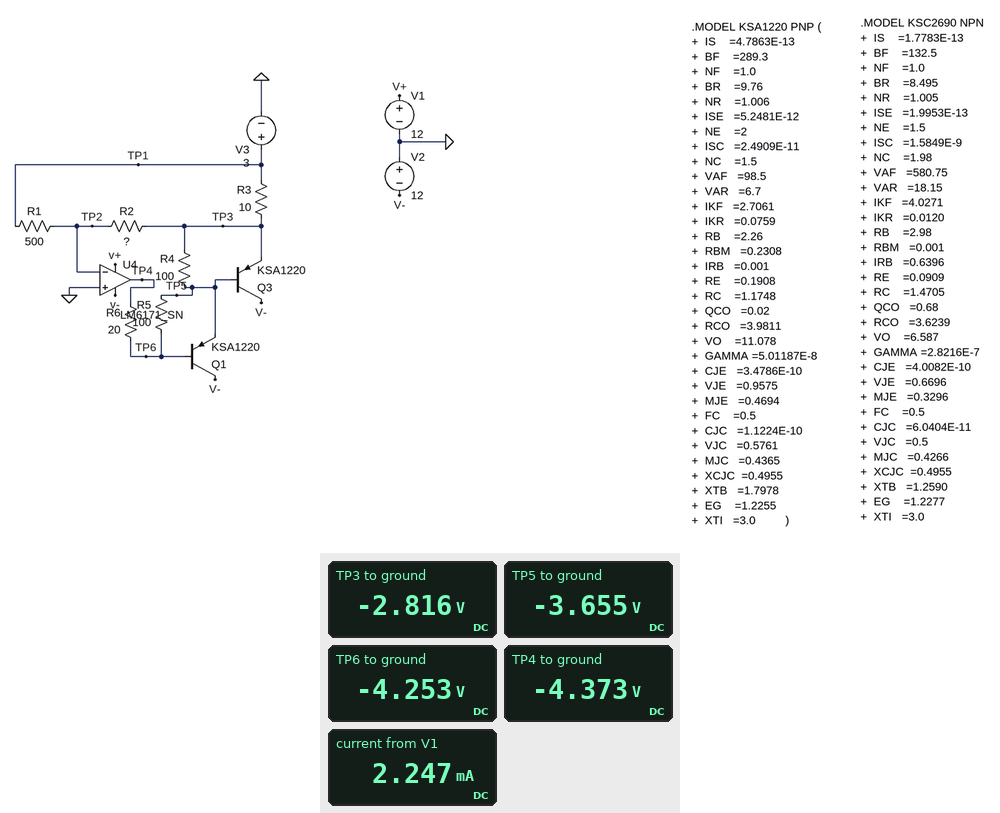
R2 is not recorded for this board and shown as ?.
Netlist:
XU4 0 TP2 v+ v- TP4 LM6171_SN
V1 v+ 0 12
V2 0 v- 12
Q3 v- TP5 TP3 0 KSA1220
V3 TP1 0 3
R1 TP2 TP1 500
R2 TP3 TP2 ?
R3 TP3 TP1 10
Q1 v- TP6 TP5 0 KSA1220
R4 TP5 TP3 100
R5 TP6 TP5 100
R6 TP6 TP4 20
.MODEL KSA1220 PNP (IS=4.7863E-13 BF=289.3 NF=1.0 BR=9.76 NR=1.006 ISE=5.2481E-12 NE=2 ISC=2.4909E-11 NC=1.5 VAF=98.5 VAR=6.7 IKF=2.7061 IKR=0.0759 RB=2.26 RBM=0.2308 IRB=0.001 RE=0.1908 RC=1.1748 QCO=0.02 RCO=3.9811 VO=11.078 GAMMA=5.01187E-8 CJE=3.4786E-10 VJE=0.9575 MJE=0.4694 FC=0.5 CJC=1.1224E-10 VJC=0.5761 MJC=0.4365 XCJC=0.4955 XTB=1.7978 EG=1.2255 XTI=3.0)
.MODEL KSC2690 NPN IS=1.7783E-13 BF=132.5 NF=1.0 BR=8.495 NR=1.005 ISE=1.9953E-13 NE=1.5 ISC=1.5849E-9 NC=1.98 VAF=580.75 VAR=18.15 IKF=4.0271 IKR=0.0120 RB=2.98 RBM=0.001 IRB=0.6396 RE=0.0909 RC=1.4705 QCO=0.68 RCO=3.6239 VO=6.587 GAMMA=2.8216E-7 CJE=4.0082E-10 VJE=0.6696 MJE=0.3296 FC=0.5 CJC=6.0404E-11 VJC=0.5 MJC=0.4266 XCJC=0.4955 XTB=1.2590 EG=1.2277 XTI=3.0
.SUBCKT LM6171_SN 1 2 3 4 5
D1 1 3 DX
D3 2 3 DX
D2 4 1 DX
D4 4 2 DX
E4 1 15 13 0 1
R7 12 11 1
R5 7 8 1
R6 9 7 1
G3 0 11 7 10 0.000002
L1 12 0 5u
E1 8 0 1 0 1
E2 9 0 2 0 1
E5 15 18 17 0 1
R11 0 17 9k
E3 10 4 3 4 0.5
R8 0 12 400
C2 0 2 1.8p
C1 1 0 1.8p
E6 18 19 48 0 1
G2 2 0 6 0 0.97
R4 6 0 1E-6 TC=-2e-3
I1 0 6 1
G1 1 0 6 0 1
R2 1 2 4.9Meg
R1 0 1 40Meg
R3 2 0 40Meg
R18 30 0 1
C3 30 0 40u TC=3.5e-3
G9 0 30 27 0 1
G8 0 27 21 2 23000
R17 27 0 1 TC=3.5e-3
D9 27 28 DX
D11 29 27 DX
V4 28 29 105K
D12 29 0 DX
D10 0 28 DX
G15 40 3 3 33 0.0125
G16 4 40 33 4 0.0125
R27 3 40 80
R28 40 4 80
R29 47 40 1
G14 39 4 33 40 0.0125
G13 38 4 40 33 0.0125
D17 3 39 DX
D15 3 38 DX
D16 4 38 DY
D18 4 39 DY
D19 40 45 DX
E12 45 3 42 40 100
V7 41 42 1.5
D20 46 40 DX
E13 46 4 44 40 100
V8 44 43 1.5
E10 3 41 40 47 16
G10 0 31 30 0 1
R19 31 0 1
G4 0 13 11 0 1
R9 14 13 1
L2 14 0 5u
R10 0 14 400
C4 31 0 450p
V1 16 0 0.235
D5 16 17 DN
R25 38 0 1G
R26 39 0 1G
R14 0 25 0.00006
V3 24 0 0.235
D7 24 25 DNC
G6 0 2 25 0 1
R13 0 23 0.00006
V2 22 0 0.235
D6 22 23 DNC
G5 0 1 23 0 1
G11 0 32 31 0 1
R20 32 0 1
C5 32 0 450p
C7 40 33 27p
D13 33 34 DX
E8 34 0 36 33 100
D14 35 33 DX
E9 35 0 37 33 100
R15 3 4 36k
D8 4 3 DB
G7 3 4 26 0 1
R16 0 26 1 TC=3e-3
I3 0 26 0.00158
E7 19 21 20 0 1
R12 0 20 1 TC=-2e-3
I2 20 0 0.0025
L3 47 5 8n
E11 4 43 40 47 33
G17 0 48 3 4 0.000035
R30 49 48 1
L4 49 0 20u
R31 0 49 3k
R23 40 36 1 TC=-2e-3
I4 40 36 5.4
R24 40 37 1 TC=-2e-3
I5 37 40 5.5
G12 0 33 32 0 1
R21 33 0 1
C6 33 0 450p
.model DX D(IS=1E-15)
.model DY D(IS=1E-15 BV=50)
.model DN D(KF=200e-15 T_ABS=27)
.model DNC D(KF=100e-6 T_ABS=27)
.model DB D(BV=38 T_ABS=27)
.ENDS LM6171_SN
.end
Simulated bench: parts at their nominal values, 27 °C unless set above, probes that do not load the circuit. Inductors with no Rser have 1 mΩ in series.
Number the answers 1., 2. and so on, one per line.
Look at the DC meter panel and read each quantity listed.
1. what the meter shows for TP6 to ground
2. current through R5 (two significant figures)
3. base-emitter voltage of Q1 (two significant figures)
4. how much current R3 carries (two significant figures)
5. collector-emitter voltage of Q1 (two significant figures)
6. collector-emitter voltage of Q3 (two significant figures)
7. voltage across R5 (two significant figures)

1. -4.253 V
2. 6.0 mA
3. -600 mV
4. 580 mA
5. -8.3 V
6. -9.2 V
7. 600 mV
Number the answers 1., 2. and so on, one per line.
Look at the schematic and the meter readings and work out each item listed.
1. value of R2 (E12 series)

1. 470 Ω
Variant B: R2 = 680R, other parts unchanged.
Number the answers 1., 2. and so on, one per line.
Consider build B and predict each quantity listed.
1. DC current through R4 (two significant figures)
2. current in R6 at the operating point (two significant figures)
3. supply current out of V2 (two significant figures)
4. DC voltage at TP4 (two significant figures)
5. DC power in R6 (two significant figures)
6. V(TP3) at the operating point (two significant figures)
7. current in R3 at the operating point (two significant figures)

1. 8.7 mA
2. 6.1 mA
3. 720 mA
4. -5.7 V
5. 730 µW
6. -4.1 V
7. 710 mA
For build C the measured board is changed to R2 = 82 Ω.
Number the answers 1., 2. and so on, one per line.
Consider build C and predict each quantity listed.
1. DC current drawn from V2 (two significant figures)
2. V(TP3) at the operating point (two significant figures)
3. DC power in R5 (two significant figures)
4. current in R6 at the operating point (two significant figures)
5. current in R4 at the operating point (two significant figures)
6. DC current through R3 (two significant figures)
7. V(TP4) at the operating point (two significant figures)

1. 360 mA
2. -490 mV
3. 3.4 mW
4. 5.9 mA
5. 7.8 mA
6. 350 mA
7. -2.0 V
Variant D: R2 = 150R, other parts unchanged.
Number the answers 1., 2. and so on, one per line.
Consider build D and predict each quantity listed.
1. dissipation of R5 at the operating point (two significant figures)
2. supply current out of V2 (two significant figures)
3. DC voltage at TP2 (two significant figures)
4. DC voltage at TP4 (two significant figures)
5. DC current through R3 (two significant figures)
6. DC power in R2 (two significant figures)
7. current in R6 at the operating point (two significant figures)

1. 3.5 mW
2. 400 mA
3. 1.8 mV
4. -2.4 V
5. 390 mA
6. 5.4 mW
7. 5.9 mA
